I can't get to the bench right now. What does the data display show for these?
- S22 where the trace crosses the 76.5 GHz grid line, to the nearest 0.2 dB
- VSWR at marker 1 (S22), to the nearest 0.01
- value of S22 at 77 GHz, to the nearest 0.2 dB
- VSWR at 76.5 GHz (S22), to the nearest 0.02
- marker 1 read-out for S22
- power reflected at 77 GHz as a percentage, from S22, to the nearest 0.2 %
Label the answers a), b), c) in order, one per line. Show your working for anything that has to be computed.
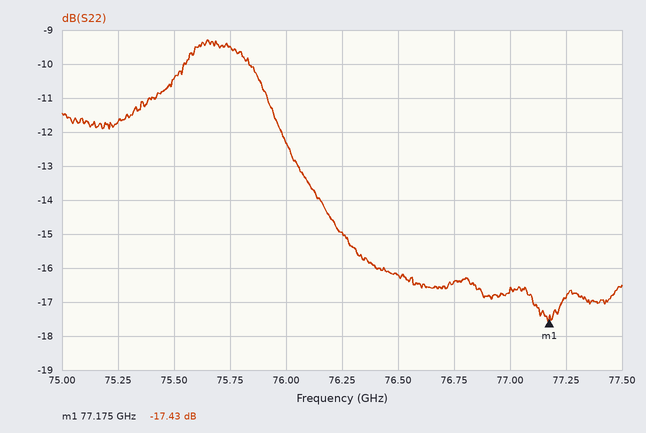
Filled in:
a) -16.2 dB
b) (1 + 0.1344)/(1 − 0.1344) ≈ 1.31
c) -16.6 dB
d) |Γ| = 10^(-16.2/20) = 0.1549; VSWR = (1 + 0.1549)/(1 − 0.1549) ≈ 1.37, so 1.36 to the nearest 0.02
e) -17.43 dB
f) 10^(-16.6/10) ≈ 2.2 %
